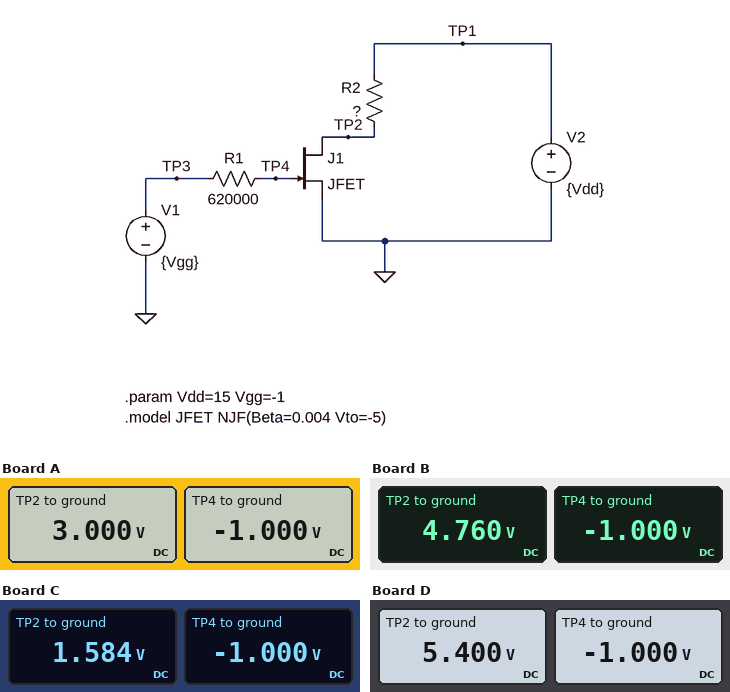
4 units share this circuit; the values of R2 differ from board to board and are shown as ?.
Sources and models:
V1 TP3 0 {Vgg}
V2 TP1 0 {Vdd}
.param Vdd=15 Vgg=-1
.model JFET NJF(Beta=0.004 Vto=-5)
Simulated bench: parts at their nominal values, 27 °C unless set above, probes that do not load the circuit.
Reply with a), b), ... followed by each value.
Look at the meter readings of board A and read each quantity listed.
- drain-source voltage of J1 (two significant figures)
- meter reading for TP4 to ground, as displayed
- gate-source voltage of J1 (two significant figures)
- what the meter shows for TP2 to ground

a) 3.0 V
b) -1.000 V
c) -1.0 V
d) 3.000 V
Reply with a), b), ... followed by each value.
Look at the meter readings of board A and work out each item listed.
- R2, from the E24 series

a) 200 Ω
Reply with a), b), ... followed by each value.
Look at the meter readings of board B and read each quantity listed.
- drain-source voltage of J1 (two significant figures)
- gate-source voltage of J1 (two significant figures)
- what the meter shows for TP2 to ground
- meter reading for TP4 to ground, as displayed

a) 4.8 V
b) -1.0 V
c) 4.760 V
d) -1.000 V
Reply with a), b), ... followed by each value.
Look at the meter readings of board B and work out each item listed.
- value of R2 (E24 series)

a) 160 Ω
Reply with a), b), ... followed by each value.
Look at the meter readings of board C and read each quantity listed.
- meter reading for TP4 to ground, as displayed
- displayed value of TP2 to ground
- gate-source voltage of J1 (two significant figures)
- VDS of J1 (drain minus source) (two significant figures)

a) -1.000 V
b) 1.584 V
c) -1.0 V
d) 1.6 V
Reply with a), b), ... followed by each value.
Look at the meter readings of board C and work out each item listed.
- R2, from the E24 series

a) 330 Ω
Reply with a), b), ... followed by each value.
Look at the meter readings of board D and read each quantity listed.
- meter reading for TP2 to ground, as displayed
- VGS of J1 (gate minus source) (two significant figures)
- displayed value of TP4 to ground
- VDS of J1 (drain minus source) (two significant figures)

a) 5.400 V
b) -1.0 V
c) -1.000 V
d) 5.4 V
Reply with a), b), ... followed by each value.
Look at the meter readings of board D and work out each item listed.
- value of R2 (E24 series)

a) 150 Ω
